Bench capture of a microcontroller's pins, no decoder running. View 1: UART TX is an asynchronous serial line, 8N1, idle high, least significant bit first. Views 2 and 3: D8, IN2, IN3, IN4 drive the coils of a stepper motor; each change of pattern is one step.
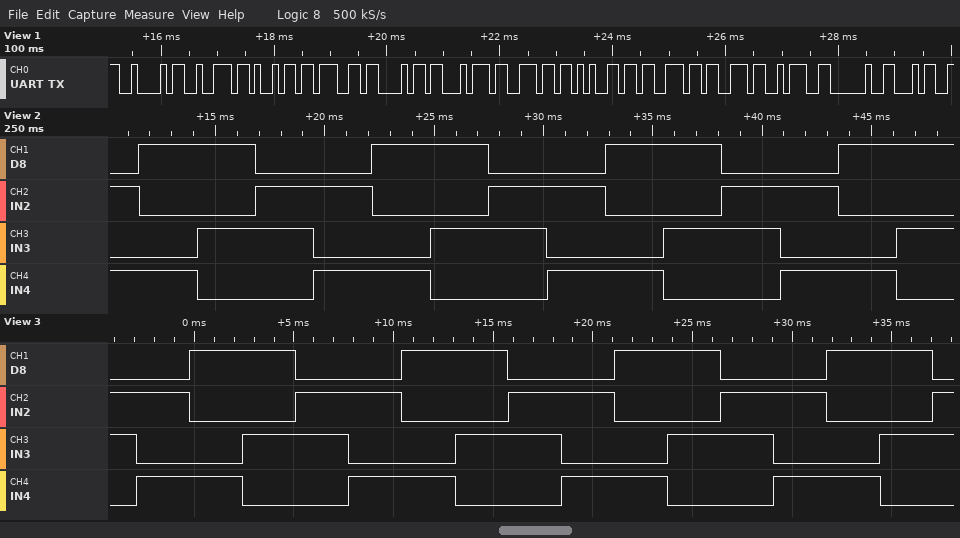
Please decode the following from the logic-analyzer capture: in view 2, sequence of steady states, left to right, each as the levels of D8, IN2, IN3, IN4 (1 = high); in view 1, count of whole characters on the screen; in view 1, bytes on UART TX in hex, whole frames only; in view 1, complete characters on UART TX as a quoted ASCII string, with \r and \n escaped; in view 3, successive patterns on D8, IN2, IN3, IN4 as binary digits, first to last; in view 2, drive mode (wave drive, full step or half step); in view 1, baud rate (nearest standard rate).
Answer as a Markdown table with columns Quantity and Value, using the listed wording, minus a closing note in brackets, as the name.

| Quantity | Value |
|---|---|
| in view 2, sequence of steady states, left to right, each as the levels of D8, IN2, IN3, IN4 | 0101 1001 1010 0110 0101 1001 1010 0110 0101 1001 1010 0110 0101 1001 1010 |
| in view 1, count of whole characters on the screen | 13 |
| in view 1, bytes on UART TX in hex, whole frames only | 42 72 69 67 68 74 6E 65 73 73 3A 20 34 |
| in view 1, complete characters on UART TX as a quoted ASCII string, with \r and \n escaped | "Brightness: 4" |
| in view 3, successive patterns on D8, IN2, IN3, IN4 as binary digits, first to last | 0110 0101 1001 1010 0110 0101 1001 1010 0110 0101 1001 1010 0110 0101 1001 1010 0110 |
| in view 2, drive mode | full step |
| in view 1, baud rate | 9600 baud |
